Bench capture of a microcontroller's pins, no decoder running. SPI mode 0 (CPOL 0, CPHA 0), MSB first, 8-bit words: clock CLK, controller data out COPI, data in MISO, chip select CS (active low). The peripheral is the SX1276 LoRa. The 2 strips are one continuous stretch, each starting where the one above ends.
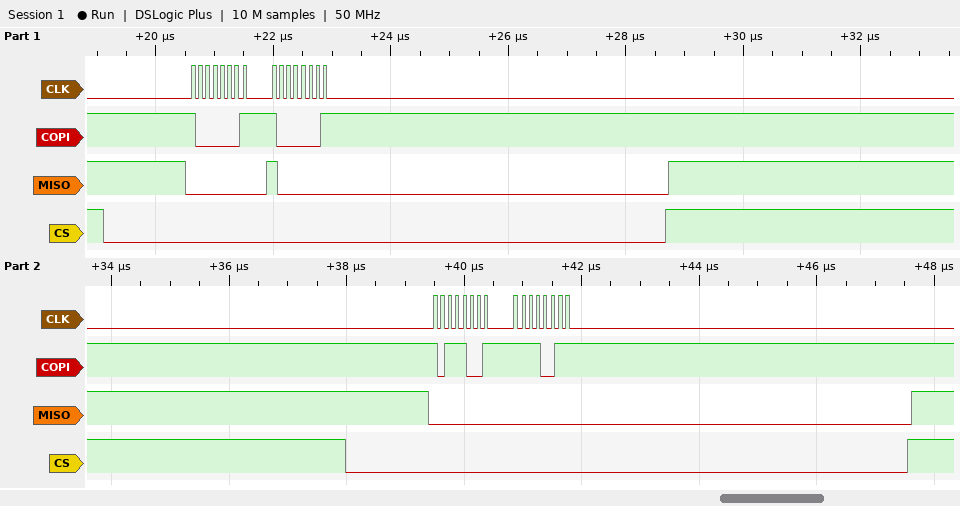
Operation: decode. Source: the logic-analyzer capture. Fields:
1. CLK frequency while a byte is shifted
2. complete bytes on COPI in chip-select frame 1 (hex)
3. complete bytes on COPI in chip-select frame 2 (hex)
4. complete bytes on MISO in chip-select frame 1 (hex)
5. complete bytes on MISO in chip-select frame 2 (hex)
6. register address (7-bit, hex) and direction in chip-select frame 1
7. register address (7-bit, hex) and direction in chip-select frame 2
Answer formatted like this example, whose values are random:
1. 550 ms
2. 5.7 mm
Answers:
1. 8 MHz
2. 81 81
3. B9 F3
4. 00 80
5. 00 00
6. 0x01 write
7. 0x39 write
